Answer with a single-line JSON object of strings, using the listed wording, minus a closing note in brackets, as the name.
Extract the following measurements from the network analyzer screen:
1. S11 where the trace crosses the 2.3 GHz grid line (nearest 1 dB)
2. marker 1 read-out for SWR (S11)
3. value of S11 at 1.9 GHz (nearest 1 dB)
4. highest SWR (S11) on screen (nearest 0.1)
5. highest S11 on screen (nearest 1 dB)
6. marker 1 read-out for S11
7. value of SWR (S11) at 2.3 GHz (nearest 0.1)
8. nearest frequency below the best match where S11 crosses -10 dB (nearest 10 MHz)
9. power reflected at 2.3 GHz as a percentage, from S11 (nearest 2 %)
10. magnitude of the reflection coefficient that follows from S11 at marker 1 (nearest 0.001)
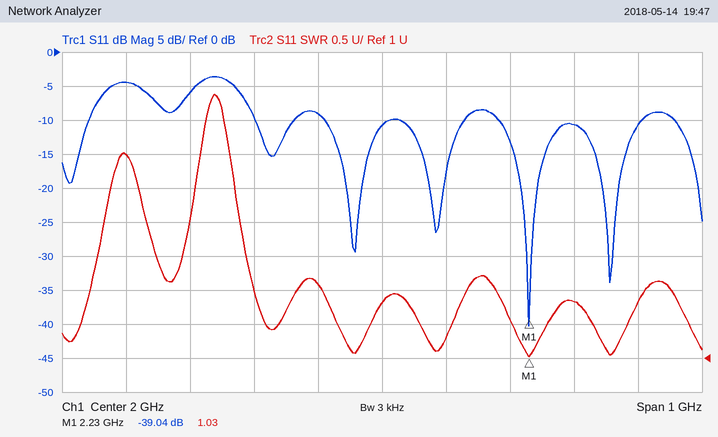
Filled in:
{"S11 where the trace crosses the 2.3 GHz grid line": "-11 dB", "marker 1 read-out for SWR": "1.03", "value of S11 at 1.9 GHz": "-9 dB", "highest SWR (S11) on screen": "4.9", "highest S11 on screen": "-4 dB", "marker 1 read-out for S11": "-39.04 dB", "value of SWR (S11) at 2.3 GHz": "1.8", "nearest frequency below the best match where S11 crosses -10 dB": "2.18 GHz", "power reflected at 2.3 GHz as a percentage, from S11": "8 %", "magnitude of the reflection coefficient that follows from S11 at marker 1": "0.011"}
